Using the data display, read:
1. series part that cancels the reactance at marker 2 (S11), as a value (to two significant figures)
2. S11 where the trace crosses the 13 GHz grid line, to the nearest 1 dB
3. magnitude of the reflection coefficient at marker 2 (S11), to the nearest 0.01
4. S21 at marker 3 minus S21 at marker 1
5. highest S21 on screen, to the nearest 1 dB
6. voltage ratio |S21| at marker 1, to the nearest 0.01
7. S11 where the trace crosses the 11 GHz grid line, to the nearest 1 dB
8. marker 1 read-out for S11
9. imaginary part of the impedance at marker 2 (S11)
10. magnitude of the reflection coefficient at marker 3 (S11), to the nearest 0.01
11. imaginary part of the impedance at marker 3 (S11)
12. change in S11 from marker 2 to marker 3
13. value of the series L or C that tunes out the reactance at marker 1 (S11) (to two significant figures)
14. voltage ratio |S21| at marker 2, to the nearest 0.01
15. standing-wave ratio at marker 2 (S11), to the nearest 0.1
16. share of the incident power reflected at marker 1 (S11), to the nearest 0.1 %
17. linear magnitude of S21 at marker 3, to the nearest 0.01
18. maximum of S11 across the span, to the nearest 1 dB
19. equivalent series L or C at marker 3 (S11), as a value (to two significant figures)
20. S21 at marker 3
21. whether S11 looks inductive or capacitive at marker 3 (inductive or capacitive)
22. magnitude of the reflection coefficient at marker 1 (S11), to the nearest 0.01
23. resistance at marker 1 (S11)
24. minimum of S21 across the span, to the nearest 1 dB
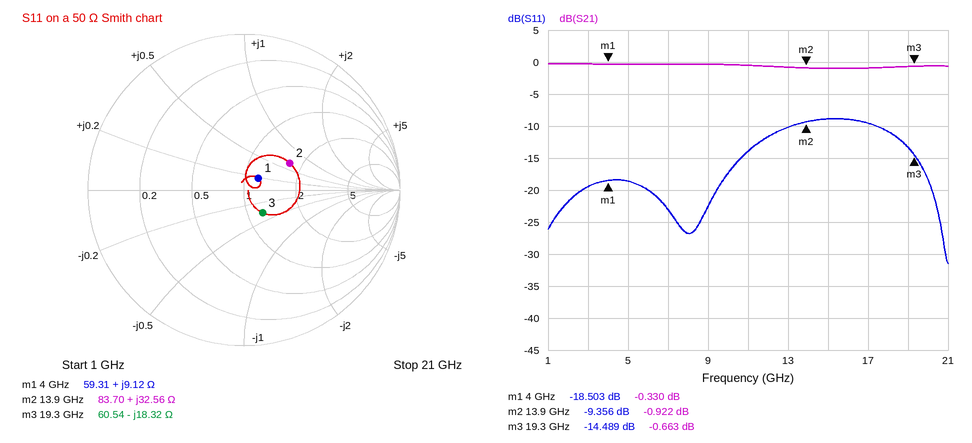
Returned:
350 fF
-10 dB
0.34
-0.333 dB
0 dB
0.96
-14 dB
-18.503 dB
+32.56 Ω
0.19
-18.32 Ω
-5.133 dB
4.4 pF
0.90
2.0
1.4 %
0.93
-9 dB
450 fF
-0.663 dB
capacitive
0.12
59.31 Ω
-1 dB
